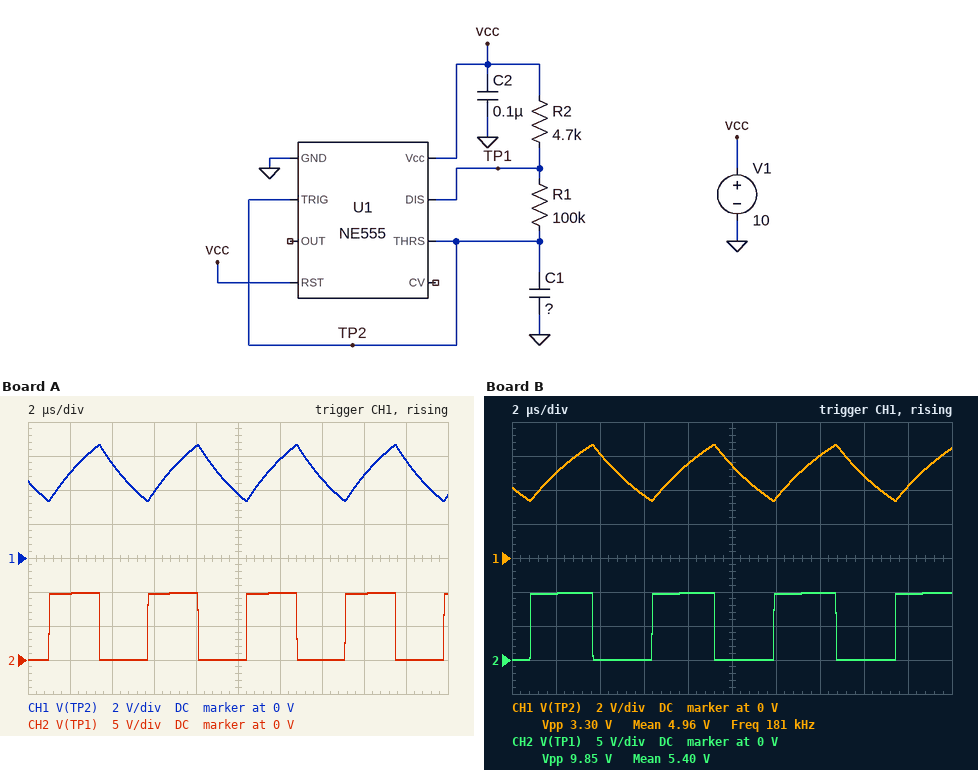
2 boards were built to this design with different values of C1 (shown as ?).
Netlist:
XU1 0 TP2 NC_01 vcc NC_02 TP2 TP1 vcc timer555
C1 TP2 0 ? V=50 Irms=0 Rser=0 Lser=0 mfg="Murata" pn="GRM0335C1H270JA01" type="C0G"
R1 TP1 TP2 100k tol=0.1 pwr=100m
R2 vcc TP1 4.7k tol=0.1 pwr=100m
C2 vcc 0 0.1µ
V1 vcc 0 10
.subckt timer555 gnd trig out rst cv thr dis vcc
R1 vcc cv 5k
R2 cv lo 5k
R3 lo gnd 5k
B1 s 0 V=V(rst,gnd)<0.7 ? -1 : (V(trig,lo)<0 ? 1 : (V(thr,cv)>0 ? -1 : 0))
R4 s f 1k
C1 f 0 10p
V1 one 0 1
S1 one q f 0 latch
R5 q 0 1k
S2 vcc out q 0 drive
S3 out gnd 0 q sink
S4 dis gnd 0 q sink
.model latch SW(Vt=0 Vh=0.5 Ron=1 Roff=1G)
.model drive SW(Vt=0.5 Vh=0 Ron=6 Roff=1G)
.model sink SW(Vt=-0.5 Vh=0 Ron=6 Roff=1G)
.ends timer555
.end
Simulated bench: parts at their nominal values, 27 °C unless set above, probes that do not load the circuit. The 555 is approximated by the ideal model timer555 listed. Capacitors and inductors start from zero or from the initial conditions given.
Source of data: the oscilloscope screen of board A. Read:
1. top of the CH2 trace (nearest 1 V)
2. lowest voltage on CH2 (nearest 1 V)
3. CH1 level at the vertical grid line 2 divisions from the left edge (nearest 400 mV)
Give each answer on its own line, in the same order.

10 V
0 V
5.6 V
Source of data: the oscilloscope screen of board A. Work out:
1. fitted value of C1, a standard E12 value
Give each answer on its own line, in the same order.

33 pF
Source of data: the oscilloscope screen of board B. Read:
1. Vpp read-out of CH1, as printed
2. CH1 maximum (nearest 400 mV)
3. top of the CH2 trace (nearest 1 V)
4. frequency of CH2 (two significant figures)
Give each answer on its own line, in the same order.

3.30 V
6.8 V
10 V
180 kHz
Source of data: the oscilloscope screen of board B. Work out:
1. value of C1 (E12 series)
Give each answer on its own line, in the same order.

39 pF
